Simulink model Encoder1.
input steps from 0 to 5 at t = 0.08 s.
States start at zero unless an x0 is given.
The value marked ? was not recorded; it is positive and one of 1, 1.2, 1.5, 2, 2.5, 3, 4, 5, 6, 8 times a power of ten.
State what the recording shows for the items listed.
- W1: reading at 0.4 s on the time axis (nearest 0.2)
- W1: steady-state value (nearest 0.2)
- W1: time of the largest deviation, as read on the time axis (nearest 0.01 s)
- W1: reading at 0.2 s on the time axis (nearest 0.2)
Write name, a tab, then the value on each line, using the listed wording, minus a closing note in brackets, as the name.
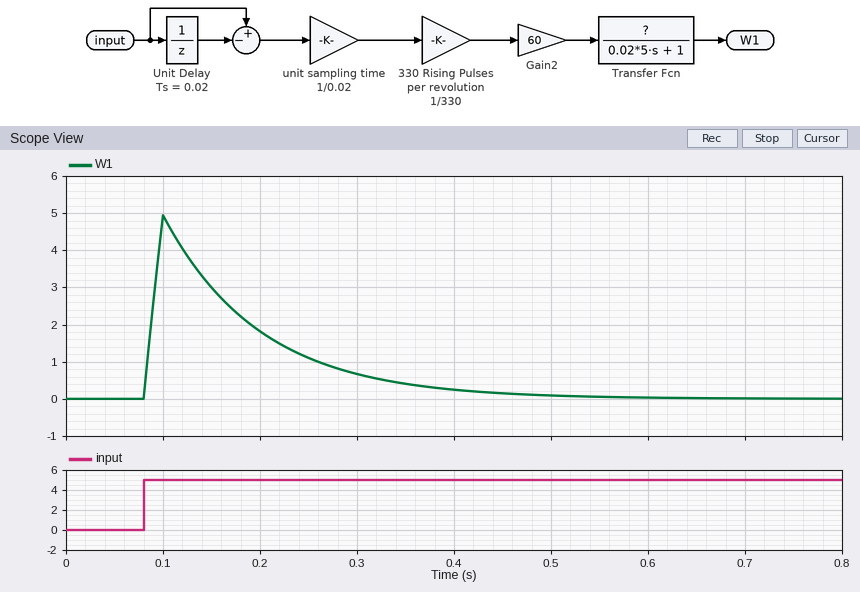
W1: reading at 0.4 s on the time axis	0.2
W1: steady-state value	0.0
W1: time of the largest deviation, as read on the time axis	0.10 s
W1: reading at 0.2 s on the time axis	1.8
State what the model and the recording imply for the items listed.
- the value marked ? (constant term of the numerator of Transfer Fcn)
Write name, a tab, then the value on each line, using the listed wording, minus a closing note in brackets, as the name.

the value marked ?	0.6
